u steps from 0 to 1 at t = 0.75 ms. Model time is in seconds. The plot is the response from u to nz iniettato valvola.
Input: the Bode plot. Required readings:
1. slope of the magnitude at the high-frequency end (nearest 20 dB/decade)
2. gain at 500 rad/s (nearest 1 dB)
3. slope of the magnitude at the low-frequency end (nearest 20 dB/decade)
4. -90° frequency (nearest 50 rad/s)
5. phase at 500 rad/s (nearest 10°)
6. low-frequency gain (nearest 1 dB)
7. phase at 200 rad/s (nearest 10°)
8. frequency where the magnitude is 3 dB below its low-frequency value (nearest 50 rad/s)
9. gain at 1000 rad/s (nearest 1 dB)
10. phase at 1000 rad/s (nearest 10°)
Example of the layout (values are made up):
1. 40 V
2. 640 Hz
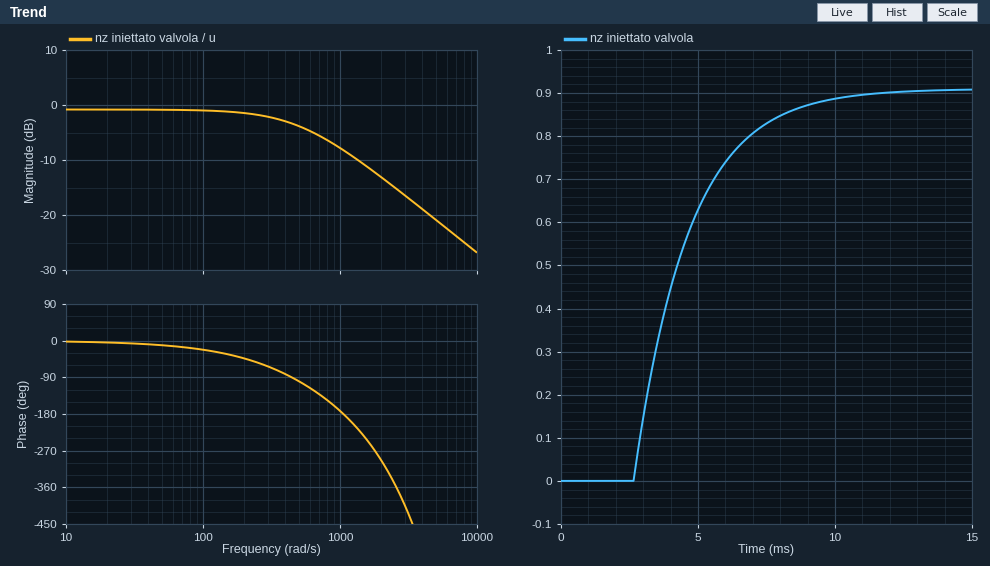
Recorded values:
1. -20 dB/decade
2. -4 dB
3. 0 dB/decade
4. 450 rad/s
5. -100°
6. -1 dB
7. -40°
8. 500 rad/s
9. -8 dB
10. -170°
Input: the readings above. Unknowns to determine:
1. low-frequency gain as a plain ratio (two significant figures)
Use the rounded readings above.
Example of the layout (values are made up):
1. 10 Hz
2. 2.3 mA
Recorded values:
1. 0.89
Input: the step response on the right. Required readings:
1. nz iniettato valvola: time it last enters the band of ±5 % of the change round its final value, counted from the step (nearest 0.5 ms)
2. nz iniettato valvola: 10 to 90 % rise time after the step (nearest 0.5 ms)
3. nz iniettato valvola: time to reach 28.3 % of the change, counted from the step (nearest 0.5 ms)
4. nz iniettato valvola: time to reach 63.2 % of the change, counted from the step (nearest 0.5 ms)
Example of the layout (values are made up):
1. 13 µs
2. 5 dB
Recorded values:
1. 8.0 ms
2. 4.5 ms
3. 2.5 ms
4. 4.0 ms
